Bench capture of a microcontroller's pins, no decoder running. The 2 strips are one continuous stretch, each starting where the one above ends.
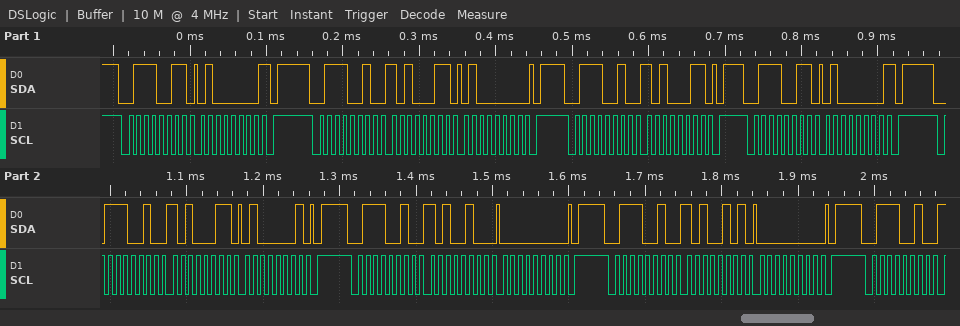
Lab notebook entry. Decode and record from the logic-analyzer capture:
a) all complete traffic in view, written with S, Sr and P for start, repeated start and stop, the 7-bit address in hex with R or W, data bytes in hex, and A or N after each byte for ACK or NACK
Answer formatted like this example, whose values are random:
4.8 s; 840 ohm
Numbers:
S 39R A 40 N P S 39W A A3 A 40 A P S 39W A A3 A P S 39R A 40 N P S 39W A A3 A 41 A P S 39W A A4 A 00 A P S 39W A A5 A 00 A P S 39W A
